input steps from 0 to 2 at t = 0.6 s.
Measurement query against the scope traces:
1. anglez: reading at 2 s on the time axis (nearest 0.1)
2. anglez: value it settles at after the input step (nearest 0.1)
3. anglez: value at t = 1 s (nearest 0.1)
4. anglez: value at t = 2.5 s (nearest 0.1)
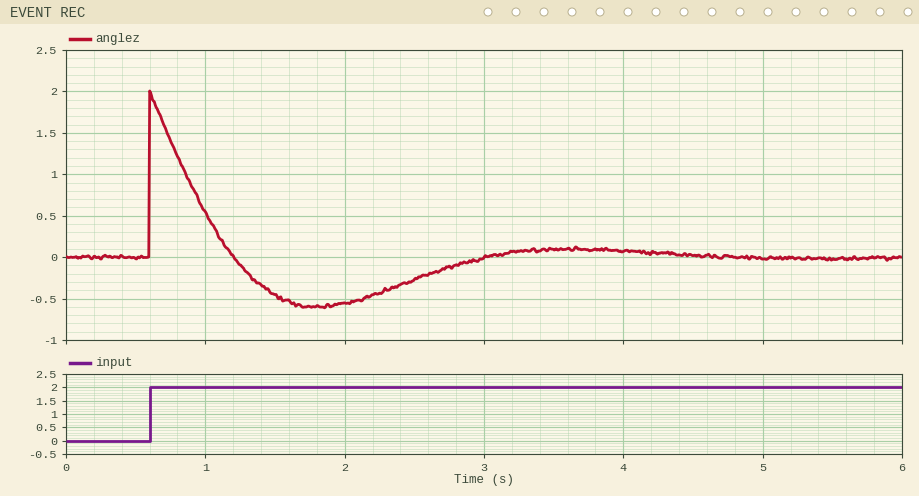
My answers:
-0.6
0.0
0.5
-0.3
